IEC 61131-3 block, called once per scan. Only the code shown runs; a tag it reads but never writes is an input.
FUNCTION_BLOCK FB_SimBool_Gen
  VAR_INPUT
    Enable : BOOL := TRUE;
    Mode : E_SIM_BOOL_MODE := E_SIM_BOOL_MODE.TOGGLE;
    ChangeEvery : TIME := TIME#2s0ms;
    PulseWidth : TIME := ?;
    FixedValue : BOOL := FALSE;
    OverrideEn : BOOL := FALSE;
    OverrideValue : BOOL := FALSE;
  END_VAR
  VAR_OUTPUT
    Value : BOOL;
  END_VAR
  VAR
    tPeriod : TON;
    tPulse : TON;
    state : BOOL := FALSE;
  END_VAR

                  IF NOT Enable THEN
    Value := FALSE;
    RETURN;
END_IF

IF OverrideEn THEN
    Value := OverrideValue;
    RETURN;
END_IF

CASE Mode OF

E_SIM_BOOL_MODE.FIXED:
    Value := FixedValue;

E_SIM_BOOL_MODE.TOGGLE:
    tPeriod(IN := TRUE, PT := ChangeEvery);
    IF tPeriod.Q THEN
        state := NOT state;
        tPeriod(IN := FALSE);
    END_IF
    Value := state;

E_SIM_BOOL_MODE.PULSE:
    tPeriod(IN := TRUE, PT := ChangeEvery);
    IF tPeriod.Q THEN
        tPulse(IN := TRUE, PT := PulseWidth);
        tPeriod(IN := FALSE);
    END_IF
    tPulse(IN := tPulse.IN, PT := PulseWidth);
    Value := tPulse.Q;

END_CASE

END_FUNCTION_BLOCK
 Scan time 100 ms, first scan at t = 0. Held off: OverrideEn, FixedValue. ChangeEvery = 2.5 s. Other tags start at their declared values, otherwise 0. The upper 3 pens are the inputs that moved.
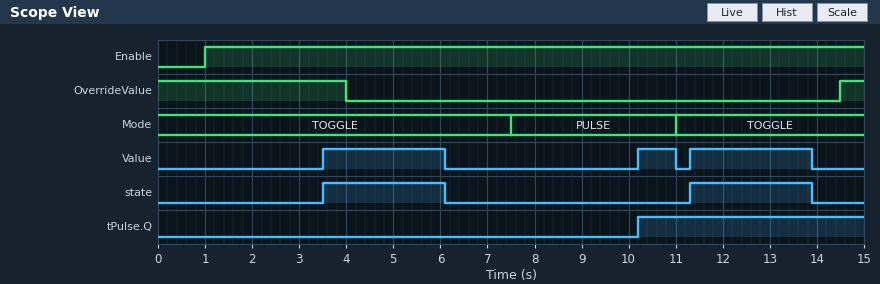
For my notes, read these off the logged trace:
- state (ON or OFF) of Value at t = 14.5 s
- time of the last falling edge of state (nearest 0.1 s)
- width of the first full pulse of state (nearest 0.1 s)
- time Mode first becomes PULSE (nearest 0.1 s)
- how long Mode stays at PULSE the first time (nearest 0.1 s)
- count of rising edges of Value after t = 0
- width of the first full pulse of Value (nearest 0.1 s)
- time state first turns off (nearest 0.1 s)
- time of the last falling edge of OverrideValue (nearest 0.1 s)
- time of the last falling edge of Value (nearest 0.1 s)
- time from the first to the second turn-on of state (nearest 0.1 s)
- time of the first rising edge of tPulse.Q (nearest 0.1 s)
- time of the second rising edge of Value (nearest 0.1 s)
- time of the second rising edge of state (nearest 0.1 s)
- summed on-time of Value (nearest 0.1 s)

OFF
13.9 s
2.6 s
7.5 s
3.5 s
3
2.6 s
6.1 s
4.0 s
13.9 s
7.8 s
10.2 s
10.2 s
11.3 s
6.0 s
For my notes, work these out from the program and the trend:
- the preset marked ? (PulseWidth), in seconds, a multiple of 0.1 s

1.5 s
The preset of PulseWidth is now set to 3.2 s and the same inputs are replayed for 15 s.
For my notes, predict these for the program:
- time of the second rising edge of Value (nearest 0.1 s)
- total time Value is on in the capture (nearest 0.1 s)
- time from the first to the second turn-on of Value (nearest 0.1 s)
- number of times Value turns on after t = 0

11.3 s
5.2 s
7.8 s
2
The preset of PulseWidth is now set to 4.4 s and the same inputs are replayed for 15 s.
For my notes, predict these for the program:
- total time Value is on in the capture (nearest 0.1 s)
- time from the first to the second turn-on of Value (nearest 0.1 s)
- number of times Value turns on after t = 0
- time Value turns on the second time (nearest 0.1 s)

5.2 s
7.8 s
2
11.3 s
